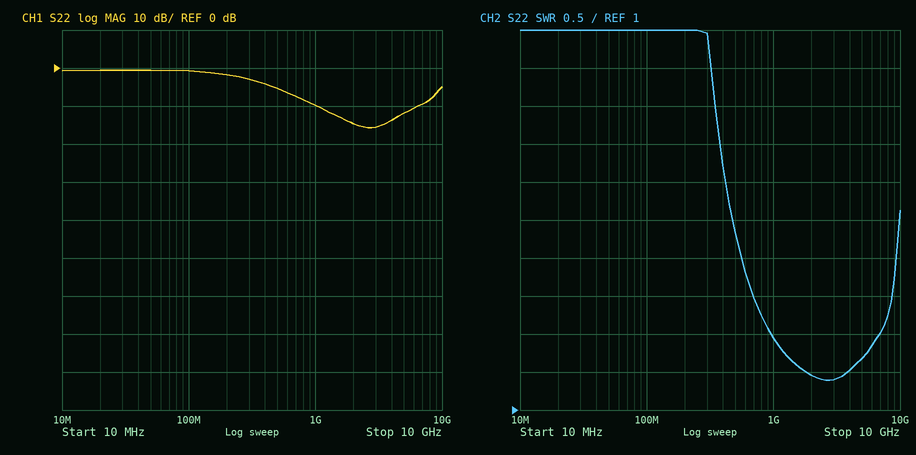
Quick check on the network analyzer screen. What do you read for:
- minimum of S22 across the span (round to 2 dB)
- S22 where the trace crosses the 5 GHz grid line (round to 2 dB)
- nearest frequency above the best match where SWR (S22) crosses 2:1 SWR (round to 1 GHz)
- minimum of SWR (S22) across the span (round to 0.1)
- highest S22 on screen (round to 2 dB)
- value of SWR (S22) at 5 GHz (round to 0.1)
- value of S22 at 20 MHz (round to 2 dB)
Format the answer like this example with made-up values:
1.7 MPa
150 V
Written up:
-16 dB
-12 dB
7 GHz
1.4
0 dB
1.7
0 dB
